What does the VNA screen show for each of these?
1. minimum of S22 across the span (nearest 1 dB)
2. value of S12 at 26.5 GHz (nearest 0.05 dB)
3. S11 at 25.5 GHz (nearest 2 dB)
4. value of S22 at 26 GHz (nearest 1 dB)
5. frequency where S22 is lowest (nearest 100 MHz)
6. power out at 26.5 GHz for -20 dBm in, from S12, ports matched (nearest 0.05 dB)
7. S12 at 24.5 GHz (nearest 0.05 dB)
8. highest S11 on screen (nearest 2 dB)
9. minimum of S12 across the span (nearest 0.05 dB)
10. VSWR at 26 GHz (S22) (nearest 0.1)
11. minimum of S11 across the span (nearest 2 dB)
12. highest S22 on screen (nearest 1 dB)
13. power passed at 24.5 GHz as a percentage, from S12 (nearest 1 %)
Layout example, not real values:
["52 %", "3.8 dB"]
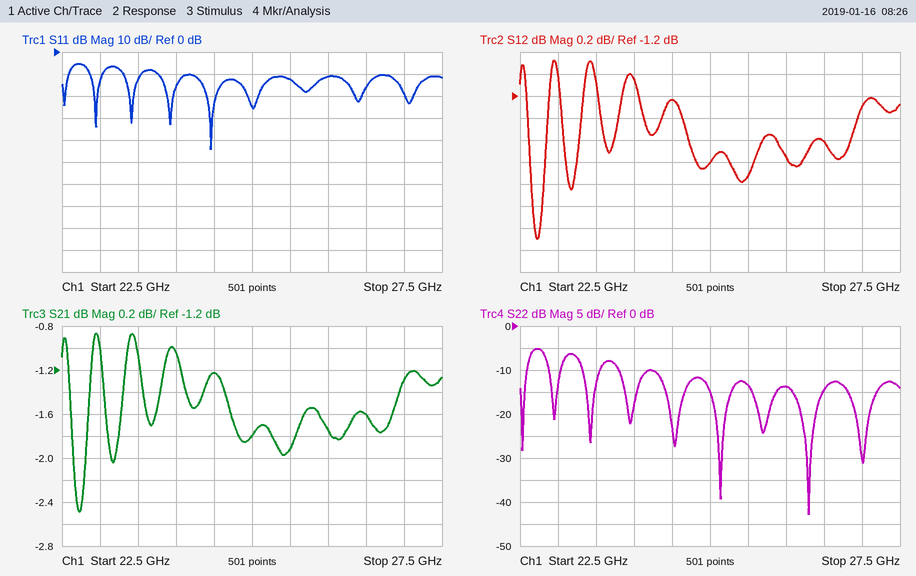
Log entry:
["-43 dB", "-1.60 dB", "-12 dB", "-14 dB", "26.3 GHz", "-21.60 dBm", "-1.25 dB", "-6 dB", "-2.50 dB", "1.5", "-44 dB", "-5 dB", "75 %"]
